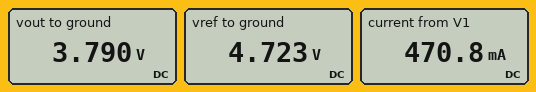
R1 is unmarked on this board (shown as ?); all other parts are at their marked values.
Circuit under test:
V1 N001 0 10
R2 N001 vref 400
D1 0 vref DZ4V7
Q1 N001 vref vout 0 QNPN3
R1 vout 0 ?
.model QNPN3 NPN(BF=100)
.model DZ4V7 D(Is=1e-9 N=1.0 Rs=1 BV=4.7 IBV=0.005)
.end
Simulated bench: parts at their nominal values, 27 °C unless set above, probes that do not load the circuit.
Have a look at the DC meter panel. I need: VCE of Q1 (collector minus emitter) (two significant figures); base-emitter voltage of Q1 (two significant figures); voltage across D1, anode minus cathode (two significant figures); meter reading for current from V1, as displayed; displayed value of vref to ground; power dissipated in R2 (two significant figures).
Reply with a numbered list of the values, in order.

1. 6.2 V
2. 930 mV
3. -4.7 V
4. 470.8 mA
5. 4.723 V
6. 70 mW
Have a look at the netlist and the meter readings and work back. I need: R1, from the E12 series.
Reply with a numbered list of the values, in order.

1. 8.2 Ω
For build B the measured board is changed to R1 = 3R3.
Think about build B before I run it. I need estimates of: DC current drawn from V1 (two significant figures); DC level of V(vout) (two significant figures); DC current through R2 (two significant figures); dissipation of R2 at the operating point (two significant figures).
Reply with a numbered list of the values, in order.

1. 1.1 A
2. 3.7 V
3. 13 mA
4. 71 mW
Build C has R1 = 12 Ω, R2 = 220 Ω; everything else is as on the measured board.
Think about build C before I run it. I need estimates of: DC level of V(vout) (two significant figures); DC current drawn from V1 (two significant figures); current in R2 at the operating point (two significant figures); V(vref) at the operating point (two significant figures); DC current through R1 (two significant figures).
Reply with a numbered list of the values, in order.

1. 3.8 V
2. 340 mA
3. 24 mA
4. 4.8 V
5. 320 mA
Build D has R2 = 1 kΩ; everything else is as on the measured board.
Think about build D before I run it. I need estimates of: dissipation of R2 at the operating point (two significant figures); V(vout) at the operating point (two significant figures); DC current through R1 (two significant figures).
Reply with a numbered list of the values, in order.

1. 29 mW
2. 3.7 V
3. 450 mA
